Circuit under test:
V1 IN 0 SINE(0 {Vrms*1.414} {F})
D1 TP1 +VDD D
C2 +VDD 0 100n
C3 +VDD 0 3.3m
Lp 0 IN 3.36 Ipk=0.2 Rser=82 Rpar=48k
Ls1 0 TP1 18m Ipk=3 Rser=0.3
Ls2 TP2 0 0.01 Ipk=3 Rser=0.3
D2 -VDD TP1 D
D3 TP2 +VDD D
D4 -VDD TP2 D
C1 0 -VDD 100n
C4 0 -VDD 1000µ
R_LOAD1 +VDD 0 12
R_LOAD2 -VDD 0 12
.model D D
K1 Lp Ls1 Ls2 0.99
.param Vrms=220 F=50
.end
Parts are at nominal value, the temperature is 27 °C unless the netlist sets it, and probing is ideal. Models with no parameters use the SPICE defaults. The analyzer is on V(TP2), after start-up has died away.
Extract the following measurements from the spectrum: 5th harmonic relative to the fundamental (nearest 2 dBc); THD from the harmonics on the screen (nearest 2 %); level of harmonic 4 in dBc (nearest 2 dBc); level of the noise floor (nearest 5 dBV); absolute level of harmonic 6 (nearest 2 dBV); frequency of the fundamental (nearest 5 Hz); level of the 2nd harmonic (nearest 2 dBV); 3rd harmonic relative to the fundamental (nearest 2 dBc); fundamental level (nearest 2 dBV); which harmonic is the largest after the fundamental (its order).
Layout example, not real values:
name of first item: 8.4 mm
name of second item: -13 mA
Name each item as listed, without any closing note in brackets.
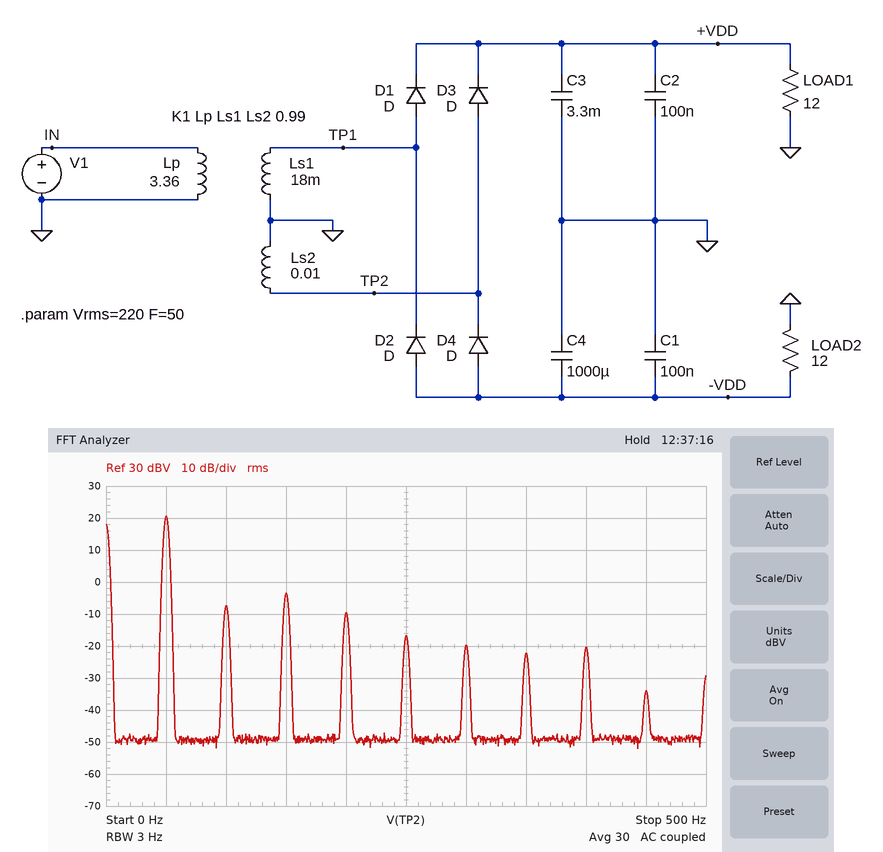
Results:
5th harmonic relative to the fundamental: -38 dBc
THD from the harmonics on the screen: 8 %
level of harmonic 4 in dBc: -30 dBc
level of the noise floor: -50 dBV
absolute level of harmonic 6: -20 dBV
frequency of the fundamental: 50 Hz
level of the 2nd harmonic: -8 dBV
3rd harmonic relative to the fundamental: -24 dBc
fundamental level: 20 dBV
which harmonic is the largest after the fundamental: 3
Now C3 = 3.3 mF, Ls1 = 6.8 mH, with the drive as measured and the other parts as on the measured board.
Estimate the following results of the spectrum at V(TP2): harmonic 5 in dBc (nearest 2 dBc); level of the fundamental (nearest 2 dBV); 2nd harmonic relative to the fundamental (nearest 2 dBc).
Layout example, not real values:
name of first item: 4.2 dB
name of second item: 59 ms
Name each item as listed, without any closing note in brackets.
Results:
harmonic 5 in dBc: -34 dBc
level of the fundamental: 20 dBV
2nd harmonic relative to the fundamental: -30 dBc
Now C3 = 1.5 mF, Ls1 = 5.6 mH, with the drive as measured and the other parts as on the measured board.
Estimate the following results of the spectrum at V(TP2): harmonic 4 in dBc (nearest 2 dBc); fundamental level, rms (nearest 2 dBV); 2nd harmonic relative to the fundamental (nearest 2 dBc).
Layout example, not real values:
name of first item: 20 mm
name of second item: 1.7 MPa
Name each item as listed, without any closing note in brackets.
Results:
harmonic 4 in dBc: -38 dBc
fundamental level, rms: 20 dBV
2nd harmonic relative to the fundamental: -38 dBc
